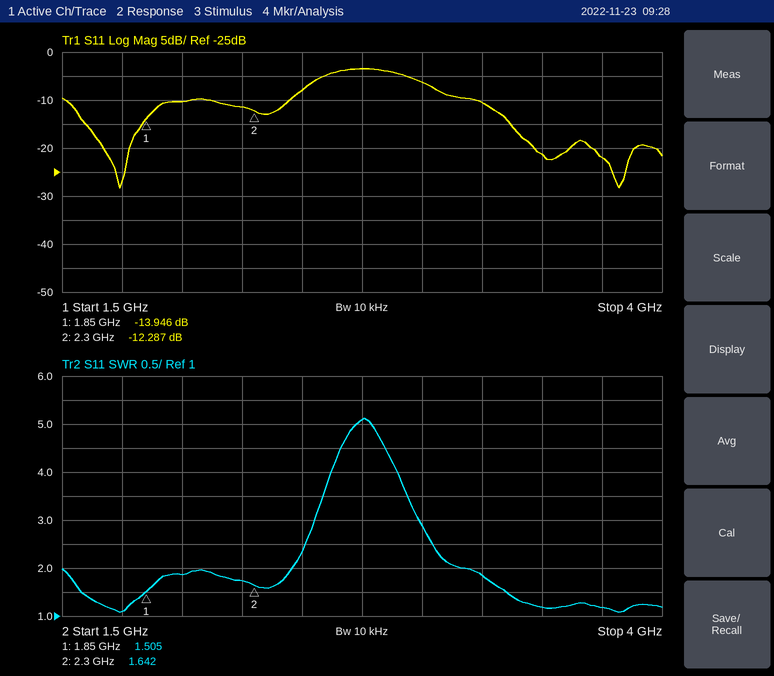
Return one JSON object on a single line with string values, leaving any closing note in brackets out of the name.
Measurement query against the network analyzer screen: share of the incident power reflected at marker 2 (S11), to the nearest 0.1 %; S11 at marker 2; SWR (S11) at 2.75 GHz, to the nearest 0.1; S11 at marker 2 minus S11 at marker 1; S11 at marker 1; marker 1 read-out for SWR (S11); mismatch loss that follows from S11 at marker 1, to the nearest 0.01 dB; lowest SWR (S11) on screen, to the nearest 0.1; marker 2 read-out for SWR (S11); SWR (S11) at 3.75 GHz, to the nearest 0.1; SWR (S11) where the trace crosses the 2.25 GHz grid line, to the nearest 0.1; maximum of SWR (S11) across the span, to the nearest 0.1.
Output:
{"share of the incident power reflected at marker 2 (S11), to the nearest 0.1 %": "5.9 %", "S11 at marker 2": "-12.287 dB", "SWR (S11) at 2.75 GHz, to the nearest 0.1": "5.1", "S11 at marker 2 minus S11 at marker 1": "1.659 dB", "S11 at marker 1": "-13.946 dB", "marker 1 read-out for SWR": "1.505", "mismatch loss that follows from S11 at marker 1, to the nearest 0.01 dB": "0.18 dB", "lowest SWR (S11) on screen, to the nearest 0.1": "1.1", "marker 2 read-out for SWR": "1.642", "SWR (S11) at 3.75 GHz, to the nearest 0.1": "1.2", "SWR (S11) where the trace crosses the 2.25 GHz grid line, to the nearest 0.1": "1.7", "maximum of SWR (S11) across the span, to the nearest 0.1": "5.1"}
